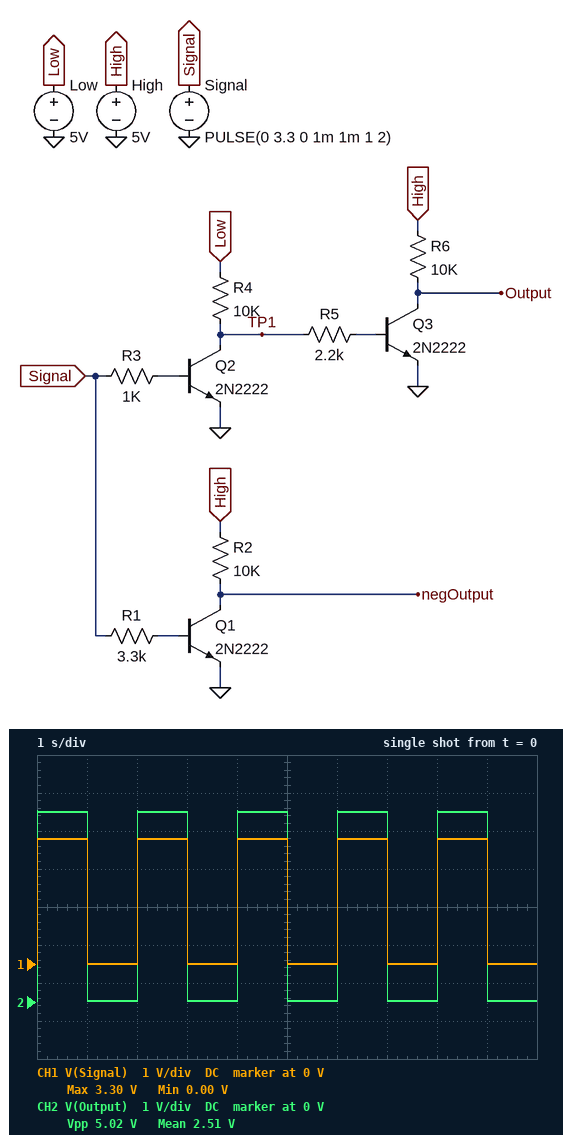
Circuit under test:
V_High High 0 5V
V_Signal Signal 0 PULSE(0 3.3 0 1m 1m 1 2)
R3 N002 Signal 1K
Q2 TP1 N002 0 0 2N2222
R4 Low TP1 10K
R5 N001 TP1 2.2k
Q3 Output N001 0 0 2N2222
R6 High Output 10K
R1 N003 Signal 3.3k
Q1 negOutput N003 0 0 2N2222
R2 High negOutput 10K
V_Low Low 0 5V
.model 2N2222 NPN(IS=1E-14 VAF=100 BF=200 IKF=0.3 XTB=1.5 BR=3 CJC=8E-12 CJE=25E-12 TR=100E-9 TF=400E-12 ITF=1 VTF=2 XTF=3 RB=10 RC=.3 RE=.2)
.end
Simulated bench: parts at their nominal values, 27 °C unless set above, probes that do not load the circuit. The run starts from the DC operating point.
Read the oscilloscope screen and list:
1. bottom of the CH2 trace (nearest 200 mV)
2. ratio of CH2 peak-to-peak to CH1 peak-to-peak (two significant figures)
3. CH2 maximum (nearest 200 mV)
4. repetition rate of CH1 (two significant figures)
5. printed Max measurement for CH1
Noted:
0 V
1.5
5.0 V
500 mHz
3.30 V
